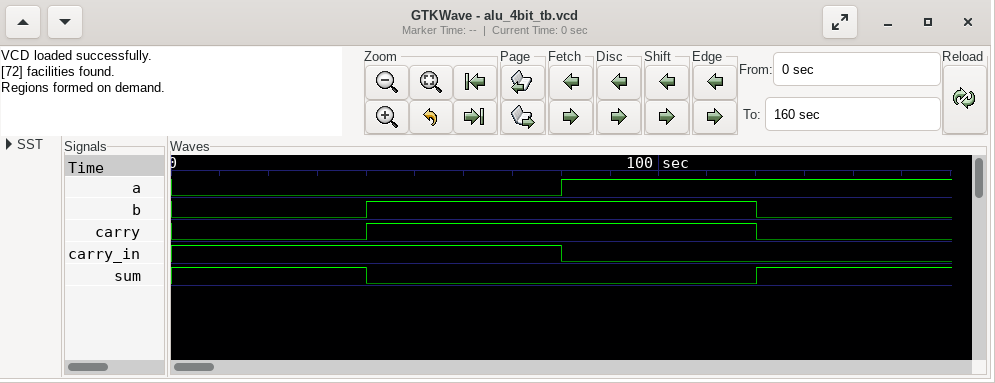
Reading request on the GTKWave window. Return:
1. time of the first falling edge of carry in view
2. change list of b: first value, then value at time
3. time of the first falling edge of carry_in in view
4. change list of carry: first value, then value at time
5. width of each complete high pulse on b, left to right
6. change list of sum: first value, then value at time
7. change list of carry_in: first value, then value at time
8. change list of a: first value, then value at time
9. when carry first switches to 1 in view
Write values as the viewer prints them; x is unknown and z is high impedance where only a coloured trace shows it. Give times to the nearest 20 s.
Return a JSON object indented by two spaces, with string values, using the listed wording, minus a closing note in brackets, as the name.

{
  "time of the first falling edge of carry in view": "120 s",
  "change list of b: first value, then value at time": "0, 1 at 40 s, 0 at 120 s",
  "time of the first falling edge of carry_in in view": "80 s",
  "change list of carry: first value, then value at time": "0, 1 at 40 s, 0 at 120 s",
  "width of each complete high pulse on b, left to right": "80 s",
  "change list of sum: first value, then value at time": "1, 0 at 40 s, 1 at 120 s",
  "change list of carry_in: first value, then value at time": "1, 0 at 80 s",
  "change list of a: first value, then value at time": "0, 1 at 80 s",
  "when carry first switches to 1 in view": "40 s"
}
